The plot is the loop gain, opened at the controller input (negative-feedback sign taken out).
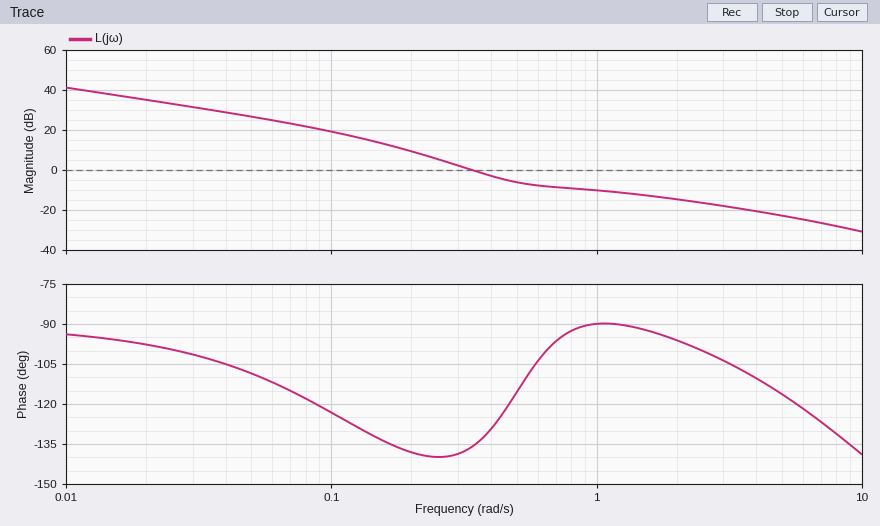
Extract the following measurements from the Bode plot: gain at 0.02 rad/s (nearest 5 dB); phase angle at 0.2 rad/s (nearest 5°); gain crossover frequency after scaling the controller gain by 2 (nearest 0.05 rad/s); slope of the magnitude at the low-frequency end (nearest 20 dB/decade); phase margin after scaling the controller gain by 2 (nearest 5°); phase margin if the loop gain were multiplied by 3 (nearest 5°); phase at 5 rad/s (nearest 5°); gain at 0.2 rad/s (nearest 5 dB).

35 dB
-140°
0.50 rad/s
-20 dB/decade
65°
90°
-115°
10 dB
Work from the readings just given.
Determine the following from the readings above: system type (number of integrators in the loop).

1
